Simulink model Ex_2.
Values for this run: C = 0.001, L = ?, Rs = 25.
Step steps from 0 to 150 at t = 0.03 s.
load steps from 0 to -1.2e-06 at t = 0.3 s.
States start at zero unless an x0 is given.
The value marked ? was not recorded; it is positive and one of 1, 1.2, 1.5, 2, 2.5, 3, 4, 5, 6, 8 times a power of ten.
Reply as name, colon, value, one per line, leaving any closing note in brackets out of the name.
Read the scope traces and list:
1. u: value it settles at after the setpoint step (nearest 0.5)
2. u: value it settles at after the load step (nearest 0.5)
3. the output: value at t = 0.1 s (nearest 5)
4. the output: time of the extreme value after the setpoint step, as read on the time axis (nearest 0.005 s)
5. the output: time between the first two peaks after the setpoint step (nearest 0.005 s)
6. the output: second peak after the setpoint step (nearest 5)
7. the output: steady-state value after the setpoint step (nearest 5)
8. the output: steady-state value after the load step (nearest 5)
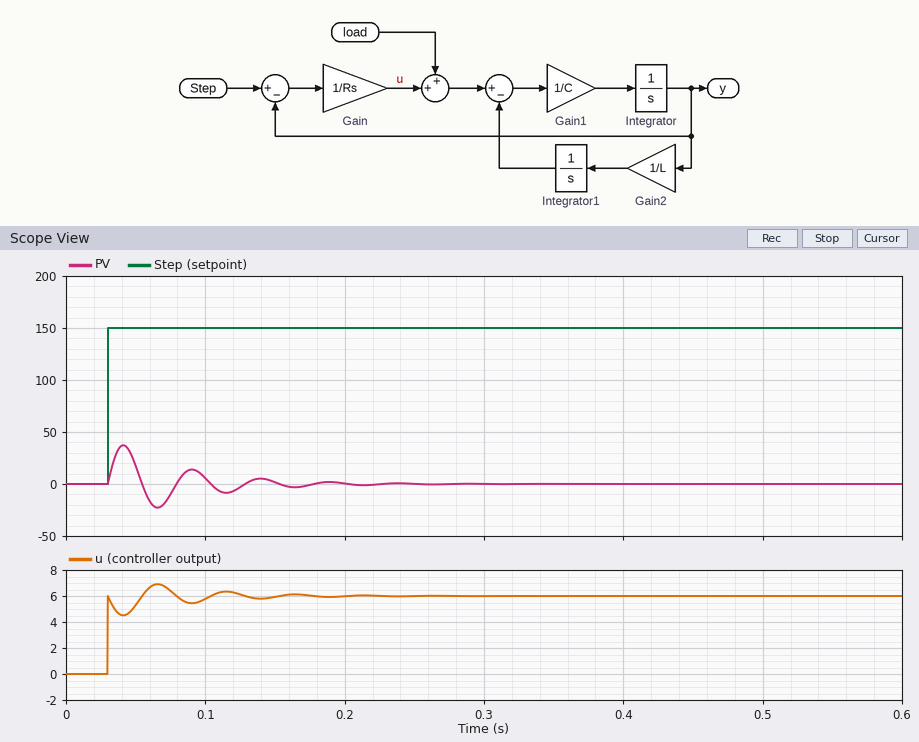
u: value it settles at after the setpoint step: 6.0
u: value it settles at after the load step: 6.0
the output: value at t = 0.1 s: 5
the output: time of the extreme value after the setpoint step, as read on the time axis: 0.040 s
the output: time between the first two peaks after the setpoint step: 0.050 s
the output: second peak after the setpoint step: 15
the output: steady-state value after the setpoint step: 0
the output: steady-state value after the load step: 0
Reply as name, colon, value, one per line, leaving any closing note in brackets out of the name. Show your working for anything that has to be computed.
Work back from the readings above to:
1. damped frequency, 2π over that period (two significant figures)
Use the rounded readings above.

damped frequency, 2π over that period: 2π / 0.05 = 130 rad/s
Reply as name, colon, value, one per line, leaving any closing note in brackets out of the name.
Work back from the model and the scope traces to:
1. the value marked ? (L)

the value marked ?: 0.06
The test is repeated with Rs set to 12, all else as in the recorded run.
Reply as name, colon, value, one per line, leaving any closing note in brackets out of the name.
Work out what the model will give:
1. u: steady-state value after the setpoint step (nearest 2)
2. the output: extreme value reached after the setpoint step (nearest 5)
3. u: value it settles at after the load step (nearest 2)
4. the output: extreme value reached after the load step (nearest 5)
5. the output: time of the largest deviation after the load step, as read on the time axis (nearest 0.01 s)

u: steady-state value after the setpoint step: 12
the output: extreme value reached after the setpoint step: 65
u: value it settles at after the load step: 12
the output: extreme value reached after the load step: 0
the output: time of the largest deviation after the load step, as read on the time axis: 0.32 s
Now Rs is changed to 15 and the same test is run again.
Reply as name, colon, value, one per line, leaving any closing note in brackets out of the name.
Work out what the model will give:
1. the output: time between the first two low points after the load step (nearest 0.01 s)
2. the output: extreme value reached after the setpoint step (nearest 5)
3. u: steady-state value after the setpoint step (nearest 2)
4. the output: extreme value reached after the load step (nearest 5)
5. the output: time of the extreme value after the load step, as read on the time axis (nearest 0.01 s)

the output: time between the first two low points after the load step: 0.05 s
the output: extreme value reached after the setpoint step: 55
u: steady-state value after the setpoint step: 10
the output: extreme value reached after the load step: 0
the output: time of the extreme value after the load step, as read on the time axis: 0.32 s
